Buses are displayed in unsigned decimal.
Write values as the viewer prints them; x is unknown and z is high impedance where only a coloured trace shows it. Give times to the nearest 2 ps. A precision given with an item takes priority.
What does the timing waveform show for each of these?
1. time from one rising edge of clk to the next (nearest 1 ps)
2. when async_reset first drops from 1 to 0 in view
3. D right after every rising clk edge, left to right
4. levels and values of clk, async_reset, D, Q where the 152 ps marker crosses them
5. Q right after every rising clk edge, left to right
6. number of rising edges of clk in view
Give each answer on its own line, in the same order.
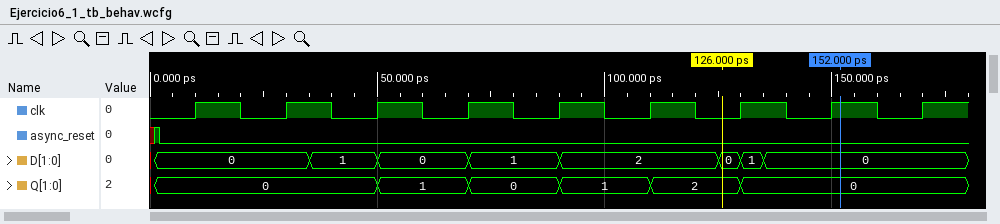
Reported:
20 ps
2 ps
0, 0, 0, 1, 2, 2, 1, 0, 0
clk=1, async_reset=0, D=0, Q=0
0, 0, 1, 0, 1, 2, 0, 0, 0
9
